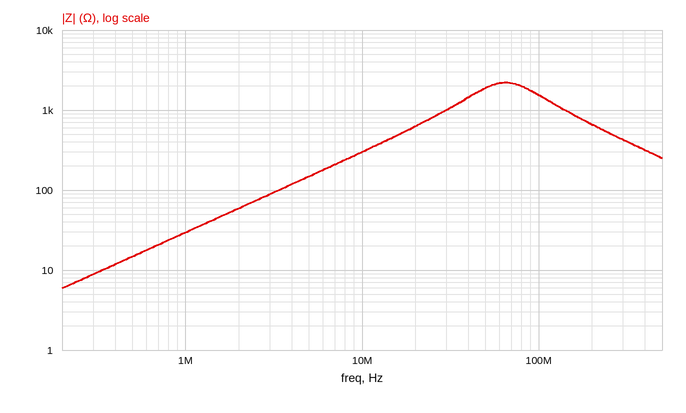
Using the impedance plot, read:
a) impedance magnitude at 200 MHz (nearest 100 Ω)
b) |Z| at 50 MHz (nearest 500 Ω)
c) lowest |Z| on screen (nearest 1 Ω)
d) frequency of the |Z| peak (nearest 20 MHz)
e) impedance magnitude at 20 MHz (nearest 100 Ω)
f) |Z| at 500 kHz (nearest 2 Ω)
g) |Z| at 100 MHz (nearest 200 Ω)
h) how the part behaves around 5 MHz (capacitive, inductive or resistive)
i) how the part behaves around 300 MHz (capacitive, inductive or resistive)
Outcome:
700 Ω
2.0 kΩ
6 Ω
60 MHz
600 Ω
14 Ω
1.6 kΩ
inductive
capacitive
